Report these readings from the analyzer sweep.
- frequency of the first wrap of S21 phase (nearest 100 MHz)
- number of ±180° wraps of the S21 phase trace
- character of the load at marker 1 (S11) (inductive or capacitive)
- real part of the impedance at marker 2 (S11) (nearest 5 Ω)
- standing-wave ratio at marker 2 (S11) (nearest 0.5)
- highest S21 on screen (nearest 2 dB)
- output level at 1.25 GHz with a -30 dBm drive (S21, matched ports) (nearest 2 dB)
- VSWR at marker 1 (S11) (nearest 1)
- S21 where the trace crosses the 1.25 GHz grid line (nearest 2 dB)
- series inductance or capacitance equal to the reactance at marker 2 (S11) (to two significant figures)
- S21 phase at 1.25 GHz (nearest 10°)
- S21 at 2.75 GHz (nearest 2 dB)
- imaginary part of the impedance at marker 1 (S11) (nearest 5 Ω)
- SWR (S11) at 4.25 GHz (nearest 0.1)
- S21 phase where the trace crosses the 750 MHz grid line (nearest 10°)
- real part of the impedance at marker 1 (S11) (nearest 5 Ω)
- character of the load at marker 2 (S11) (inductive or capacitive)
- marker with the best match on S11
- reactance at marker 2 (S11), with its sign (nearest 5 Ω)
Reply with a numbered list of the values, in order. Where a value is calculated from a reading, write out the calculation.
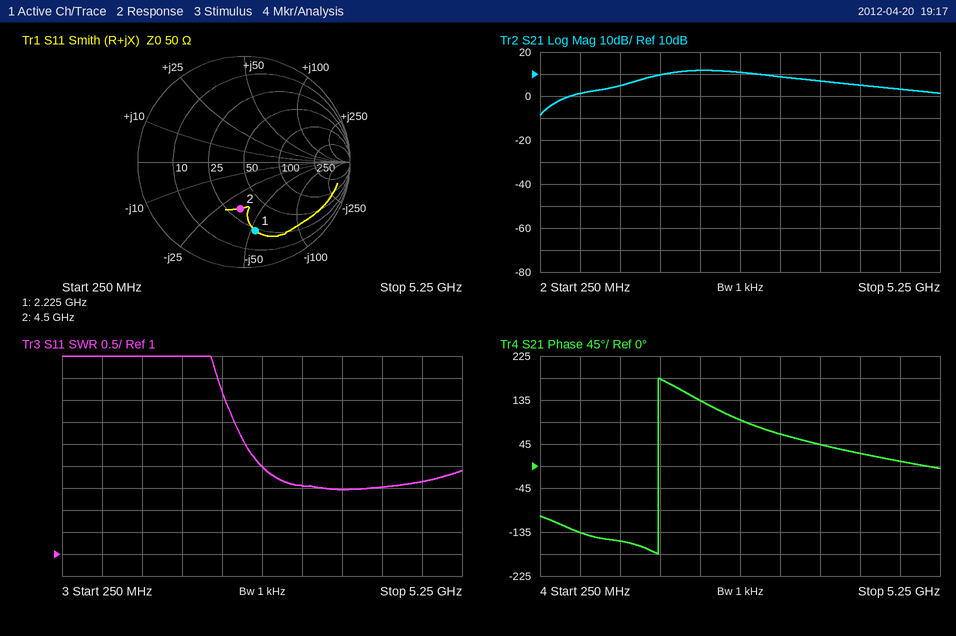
1. 1.7 GHz
2. 1
3. capacitive
4. 30 Ω
5. 2.5
6. 12 dB
7. -30 dBm + (4 dB) = -26 dBm
8. 5
9. 4 dB
10. C = 1/(2π × 4.5 GHz × 35 Ω) ≈ 1.0 pF
11. -150°
12. 10 dB
13. -55 Ω
14. 2.5
15. -140°
16. 25 Ω
17. capacitive
18. marker 2
19. -35 Ω
